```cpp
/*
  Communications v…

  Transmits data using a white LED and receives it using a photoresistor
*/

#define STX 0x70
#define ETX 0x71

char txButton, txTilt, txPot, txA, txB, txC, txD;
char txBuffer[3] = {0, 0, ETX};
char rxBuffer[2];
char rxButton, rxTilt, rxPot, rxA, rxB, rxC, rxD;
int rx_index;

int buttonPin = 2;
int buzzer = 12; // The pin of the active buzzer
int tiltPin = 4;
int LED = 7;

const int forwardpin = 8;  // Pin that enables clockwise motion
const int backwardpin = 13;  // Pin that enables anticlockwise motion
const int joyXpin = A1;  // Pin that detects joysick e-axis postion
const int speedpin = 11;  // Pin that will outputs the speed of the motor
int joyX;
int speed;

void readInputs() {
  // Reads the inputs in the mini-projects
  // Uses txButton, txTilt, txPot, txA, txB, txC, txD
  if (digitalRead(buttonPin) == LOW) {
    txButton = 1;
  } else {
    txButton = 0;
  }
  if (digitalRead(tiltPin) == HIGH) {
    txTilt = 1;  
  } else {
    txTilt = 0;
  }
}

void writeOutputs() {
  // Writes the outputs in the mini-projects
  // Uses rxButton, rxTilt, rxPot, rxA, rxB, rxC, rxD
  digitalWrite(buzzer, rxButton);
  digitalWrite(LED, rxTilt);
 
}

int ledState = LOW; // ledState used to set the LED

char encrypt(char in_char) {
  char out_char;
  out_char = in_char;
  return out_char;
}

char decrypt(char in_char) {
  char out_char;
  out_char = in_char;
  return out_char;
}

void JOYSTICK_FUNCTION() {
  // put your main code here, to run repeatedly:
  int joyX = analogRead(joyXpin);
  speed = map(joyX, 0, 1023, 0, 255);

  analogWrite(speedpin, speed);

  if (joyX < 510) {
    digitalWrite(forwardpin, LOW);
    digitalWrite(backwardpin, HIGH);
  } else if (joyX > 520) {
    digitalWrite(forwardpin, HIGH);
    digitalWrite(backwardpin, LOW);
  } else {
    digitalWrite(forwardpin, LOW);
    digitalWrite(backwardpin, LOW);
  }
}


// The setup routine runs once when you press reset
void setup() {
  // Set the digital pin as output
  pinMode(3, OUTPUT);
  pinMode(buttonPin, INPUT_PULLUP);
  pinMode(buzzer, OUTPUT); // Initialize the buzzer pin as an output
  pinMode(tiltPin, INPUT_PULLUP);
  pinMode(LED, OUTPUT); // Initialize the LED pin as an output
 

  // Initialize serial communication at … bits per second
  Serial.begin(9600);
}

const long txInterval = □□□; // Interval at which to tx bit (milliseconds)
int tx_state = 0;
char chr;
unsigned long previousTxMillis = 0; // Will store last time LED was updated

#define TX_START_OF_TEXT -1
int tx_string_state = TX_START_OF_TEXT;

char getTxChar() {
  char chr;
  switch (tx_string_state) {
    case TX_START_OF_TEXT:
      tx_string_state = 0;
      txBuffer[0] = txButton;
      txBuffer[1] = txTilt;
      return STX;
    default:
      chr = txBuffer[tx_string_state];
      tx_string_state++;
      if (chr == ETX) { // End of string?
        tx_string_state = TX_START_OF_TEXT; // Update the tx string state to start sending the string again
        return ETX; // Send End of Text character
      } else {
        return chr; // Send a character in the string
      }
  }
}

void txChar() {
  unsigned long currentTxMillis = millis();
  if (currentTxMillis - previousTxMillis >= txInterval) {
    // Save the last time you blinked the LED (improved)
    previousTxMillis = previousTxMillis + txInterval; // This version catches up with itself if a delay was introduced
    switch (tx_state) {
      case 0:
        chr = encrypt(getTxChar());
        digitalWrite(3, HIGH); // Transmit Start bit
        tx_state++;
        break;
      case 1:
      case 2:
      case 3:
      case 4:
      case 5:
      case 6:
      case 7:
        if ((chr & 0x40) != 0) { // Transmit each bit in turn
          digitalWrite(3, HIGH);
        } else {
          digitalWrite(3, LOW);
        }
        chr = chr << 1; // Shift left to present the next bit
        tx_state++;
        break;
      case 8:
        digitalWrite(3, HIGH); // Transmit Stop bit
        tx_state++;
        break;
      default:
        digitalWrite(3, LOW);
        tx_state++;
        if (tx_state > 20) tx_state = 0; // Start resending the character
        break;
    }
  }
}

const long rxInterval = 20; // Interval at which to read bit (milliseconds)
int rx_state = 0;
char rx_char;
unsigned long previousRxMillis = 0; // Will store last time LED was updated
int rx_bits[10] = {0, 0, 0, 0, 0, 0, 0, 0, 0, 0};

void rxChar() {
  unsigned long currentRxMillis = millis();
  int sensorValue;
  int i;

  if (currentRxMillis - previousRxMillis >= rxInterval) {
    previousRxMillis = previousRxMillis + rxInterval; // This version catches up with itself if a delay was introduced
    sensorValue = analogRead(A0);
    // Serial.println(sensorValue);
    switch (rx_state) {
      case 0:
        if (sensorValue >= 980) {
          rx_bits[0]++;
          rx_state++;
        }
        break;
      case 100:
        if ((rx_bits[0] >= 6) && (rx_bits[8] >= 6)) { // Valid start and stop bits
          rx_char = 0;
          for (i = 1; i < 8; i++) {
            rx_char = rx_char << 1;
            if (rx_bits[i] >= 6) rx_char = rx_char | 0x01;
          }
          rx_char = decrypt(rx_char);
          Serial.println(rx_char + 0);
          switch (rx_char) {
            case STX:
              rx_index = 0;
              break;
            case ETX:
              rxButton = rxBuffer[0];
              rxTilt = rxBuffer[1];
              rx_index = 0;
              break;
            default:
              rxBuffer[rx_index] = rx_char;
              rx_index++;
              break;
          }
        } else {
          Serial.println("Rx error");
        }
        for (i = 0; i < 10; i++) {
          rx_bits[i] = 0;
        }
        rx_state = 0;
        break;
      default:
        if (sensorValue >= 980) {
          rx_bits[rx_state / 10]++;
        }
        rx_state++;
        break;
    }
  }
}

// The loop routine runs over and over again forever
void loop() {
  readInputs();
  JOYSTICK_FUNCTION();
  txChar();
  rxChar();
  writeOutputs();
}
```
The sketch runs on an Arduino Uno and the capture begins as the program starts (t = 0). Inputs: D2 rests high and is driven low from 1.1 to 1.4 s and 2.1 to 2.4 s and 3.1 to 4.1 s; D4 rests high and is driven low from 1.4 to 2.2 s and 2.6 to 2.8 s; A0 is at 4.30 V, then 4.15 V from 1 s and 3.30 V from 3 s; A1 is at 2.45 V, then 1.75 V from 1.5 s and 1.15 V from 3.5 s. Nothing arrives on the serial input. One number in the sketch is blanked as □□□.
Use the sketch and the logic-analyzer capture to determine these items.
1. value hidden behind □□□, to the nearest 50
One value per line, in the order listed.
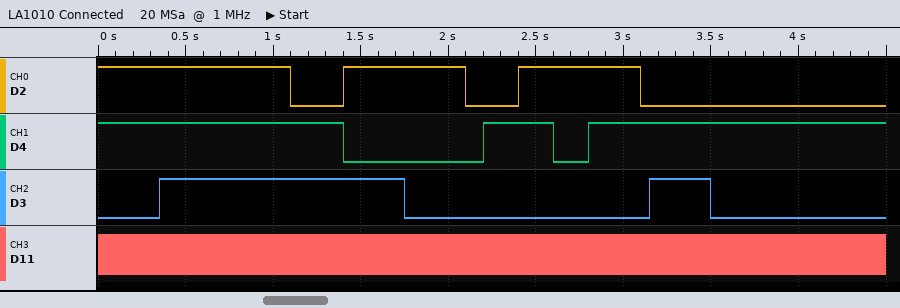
350
